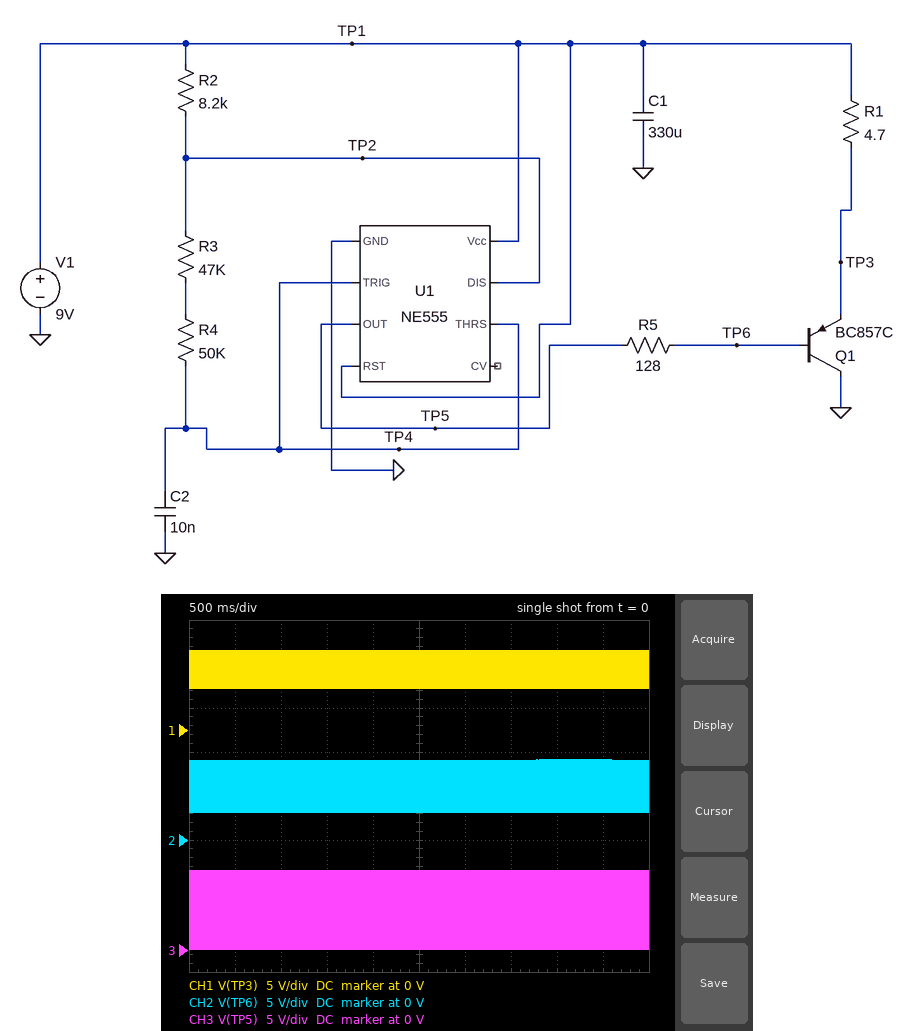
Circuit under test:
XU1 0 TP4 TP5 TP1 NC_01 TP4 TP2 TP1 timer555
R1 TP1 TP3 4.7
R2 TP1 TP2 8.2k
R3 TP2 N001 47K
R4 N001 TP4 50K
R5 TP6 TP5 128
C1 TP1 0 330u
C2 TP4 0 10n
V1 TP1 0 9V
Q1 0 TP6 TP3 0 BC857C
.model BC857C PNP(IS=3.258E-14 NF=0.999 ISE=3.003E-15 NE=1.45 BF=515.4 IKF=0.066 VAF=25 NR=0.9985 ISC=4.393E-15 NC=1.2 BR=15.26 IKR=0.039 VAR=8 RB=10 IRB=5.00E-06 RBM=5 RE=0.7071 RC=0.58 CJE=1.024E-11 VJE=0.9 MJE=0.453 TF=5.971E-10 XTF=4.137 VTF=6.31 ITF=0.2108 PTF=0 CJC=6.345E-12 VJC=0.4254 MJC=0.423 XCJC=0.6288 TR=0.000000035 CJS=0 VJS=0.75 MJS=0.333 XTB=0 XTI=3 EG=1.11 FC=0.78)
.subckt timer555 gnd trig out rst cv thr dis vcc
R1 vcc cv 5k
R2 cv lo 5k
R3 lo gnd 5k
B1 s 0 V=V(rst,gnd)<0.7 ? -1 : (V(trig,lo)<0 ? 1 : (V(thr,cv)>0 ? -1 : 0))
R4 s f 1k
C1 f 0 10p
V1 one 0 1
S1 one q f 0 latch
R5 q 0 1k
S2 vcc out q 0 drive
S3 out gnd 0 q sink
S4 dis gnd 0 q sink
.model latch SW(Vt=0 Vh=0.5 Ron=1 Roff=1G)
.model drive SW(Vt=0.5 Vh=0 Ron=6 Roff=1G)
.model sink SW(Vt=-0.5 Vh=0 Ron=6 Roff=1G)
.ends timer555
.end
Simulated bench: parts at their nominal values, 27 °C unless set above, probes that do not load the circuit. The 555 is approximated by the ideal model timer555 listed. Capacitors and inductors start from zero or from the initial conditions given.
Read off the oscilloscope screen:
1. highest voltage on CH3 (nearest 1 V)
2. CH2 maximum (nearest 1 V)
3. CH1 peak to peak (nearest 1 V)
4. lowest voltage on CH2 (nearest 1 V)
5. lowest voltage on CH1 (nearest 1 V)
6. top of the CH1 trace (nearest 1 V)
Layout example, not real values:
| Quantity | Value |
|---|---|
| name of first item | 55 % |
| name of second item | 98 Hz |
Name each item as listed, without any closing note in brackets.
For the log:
| Quantity | Value |
|---|---|
| highest voltage on CH3 | 9 V |
| CH2 maximum | 9 V |
| CH1 peak to peak | 4 V |
| lowest voltage on CH2 | 3 V |
| lowest voltage on CH1 | 5 V |
| top of the CH1 trace | 9 V |
